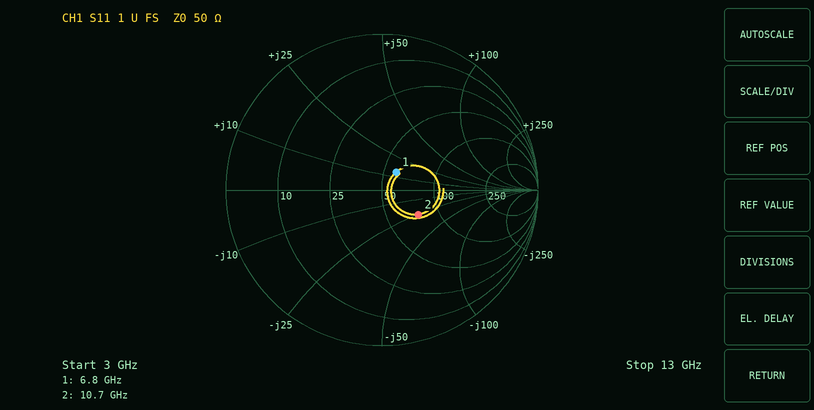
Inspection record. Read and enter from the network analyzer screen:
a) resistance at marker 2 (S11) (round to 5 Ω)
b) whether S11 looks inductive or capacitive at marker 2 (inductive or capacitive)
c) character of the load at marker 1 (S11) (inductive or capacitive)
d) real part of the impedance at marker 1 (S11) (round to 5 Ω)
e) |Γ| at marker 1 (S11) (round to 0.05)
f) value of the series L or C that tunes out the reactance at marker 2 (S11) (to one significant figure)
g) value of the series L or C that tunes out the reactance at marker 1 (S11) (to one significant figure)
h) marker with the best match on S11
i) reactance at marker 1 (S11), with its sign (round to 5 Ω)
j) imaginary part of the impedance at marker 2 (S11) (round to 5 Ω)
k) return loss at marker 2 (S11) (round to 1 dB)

75 Ω
capacitive
inductive
60 Ω
0.15
400 pH
2 pF
marker 1
+15 Ω
-25 Ω
11 dB
